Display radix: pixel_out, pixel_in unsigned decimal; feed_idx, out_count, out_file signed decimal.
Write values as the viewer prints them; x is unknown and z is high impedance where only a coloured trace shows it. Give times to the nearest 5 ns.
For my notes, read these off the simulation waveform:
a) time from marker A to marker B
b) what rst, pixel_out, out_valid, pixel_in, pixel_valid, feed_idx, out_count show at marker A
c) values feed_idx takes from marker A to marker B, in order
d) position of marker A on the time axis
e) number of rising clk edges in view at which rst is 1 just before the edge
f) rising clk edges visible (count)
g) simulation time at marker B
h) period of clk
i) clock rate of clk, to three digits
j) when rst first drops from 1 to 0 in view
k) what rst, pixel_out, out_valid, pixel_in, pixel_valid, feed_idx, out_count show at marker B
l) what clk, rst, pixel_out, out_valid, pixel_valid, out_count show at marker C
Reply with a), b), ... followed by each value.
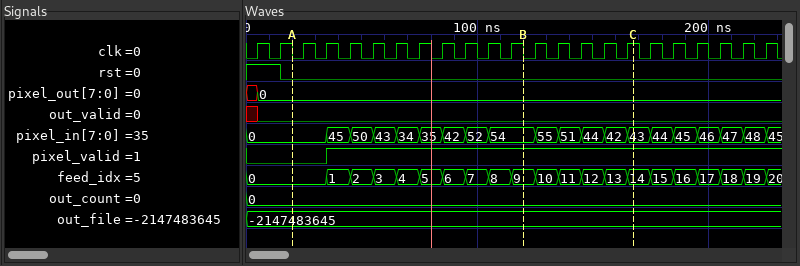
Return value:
a) 100 ns
b) rst=0, pixel_out=0, out_valid=0, pixel_in=0, pixel_valid=0, feed_idx=0, out_count=0
c) 0, 1, 2, 3, 4, 5, 6, 7, 8, 9
d) 20 ns
e) 2
f) 23
g) 120 ns
h) 10 ns
i) 100 MHz
j) 15 ns
k) rst=0, pixel_out=0, out_valid=0, pixel_in=54, pixel_valid=1, feed_idx=9, out_count=0
l) clk=1, rst=0, pixel_out=0, out_valid=0, pixel_valid=1, out_count=0
